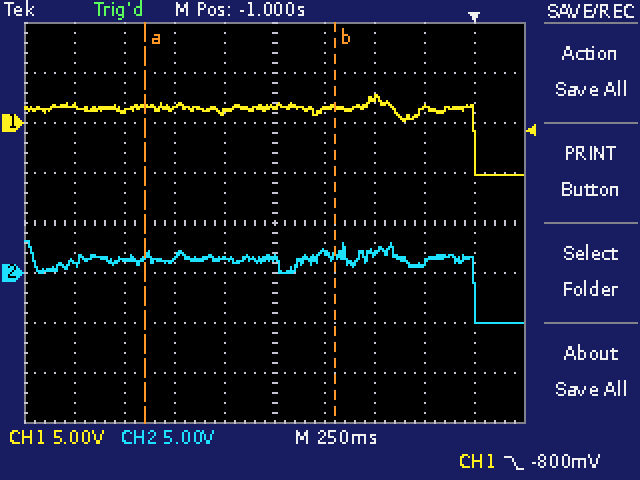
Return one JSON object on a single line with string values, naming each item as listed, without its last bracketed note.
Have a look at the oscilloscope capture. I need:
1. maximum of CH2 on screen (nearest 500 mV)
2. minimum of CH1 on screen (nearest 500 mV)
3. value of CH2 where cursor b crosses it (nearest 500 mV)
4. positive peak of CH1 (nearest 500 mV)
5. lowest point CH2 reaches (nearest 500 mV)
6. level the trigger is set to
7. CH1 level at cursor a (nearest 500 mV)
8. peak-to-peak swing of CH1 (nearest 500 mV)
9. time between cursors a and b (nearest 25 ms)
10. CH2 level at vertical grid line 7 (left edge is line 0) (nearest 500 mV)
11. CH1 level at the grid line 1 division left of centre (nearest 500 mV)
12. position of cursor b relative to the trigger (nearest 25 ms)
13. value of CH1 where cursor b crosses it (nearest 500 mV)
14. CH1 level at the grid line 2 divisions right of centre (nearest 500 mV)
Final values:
{"maximum of CH2 on screen": "3.0 V", "minimum of CH1 on screen": "-5.0 V", "value of CH2 where cursor b crosses it": "1.5 V", "positive peak of CH1": "3.0 V", "lowest point CH2 reaches": "-5.0 V", "level the trigger is set to": "-800 mV", "CH1 level at cursor a": "1.5 V", "peak-to-peak swing of CH1": "8.0 V", "time between cursors a and b": "950 ms", "CH2 level at vertical grid line 7 (left edge is line 0)": "2.0 V", "CH1 level at the grid line 1 division left of centre": "1.0 V", "position of cursor b relative to the trigger": "-700 ms", "value of CH1 where cursor b crosses it": "1.5 V", "CH1 level at the grid line 2 divisions right of centre": "2.5 V"}
